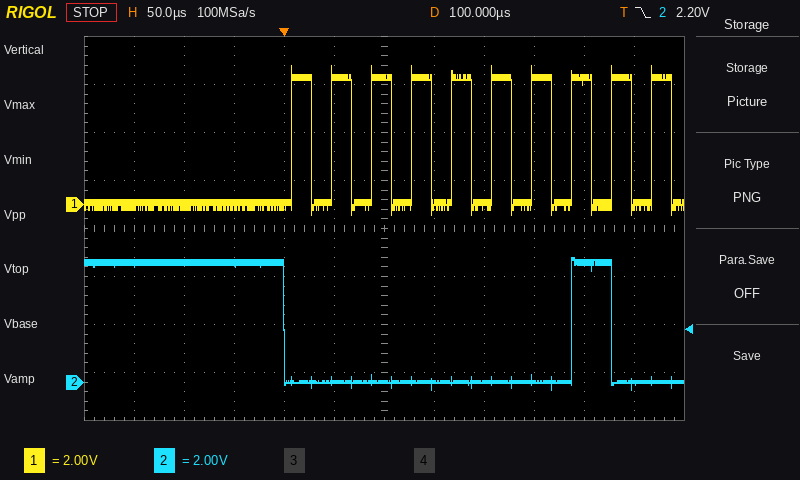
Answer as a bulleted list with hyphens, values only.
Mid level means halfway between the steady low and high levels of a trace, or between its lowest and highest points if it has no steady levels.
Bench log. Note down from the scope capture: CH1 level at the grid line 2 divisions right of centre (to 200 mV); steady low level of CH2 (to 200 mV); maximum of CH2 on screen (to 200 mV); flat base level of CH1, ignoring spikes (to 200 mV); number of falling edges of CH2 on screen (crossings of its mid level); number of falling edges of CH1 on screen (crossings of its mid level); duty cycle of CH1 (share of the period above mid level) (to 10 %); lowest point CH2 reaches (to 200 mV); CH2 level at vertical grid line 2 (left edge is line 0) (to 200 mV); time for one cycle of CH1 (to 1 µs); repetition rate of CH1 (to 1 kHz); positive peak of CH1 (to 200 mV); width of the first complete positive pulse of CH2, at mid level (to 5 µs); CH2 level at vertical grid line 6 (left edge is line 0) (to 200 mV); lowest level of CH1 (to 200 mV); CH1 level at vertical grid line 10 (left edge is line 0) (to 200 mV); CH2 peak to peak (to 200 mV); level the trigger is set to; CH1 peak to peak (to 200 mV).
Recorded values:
- 0.0 V
- 0.0 V
- 5.2 V
- 0.0 V
- 2
- 10
- 50 %
- -400 mV
- 5.0 V
- 40 µs
- 25 kHz
- 5.8 V
- 40 µs
- 0.0 V
- -400 mV
- 5.2 V
- 5.6 V
- 2.20 V
- 6.2 V
